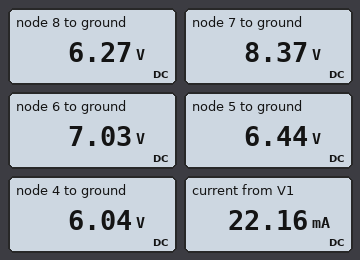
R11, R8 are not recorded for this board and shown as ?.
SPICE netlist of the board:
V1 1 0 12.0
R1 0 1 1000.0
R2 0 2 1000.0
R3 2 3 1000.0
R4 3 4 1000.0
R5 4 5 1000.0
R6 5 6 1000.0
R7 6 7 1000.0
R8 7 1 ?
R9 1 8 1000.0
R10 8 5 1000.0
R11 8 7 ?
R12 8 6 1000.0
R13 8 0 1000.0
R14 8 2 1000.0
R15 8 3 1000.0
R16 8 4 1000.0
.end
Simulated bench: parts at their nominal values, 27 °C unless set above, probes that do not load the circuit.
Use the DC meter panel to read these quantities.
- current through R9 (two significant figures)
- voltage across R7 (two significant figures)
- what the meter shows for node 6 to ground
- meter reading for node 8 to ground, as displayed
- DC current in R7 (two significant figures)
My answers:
5.7 mA
1.3 V
7.03 V
6.27 V
1.3 mA
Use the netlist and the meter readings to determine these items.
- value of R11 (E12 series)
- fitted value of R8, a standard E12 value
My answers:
680 Ω
820 Ω
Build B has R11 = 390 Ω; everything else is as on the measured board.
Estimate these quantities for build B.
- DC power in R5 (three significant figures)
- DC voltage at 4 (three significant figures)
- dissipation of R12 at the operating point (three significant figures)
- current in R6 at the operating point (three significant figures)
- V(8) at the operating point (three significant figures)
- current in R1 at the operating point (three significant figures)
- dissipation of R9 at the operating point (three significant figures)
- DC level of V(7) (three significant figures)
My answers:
131 µW
6.18 V
290 µW
450 µA
6.45 V
12.0 mA
30.8 mW
7.98 V
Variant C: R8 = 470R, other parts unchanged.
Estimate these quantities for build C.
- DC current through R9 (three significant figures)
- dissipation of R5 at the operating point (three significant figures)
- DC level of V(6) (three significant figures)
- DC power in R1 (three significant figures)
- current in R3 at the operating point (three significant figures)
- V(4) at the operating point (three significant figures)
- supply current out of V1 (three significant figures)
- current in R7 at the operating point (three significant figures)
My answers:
5.29 mA
224 µW
7.68 V
144 mW
1.62 mA
6.49 V
22.9 mA
1.69 mA
